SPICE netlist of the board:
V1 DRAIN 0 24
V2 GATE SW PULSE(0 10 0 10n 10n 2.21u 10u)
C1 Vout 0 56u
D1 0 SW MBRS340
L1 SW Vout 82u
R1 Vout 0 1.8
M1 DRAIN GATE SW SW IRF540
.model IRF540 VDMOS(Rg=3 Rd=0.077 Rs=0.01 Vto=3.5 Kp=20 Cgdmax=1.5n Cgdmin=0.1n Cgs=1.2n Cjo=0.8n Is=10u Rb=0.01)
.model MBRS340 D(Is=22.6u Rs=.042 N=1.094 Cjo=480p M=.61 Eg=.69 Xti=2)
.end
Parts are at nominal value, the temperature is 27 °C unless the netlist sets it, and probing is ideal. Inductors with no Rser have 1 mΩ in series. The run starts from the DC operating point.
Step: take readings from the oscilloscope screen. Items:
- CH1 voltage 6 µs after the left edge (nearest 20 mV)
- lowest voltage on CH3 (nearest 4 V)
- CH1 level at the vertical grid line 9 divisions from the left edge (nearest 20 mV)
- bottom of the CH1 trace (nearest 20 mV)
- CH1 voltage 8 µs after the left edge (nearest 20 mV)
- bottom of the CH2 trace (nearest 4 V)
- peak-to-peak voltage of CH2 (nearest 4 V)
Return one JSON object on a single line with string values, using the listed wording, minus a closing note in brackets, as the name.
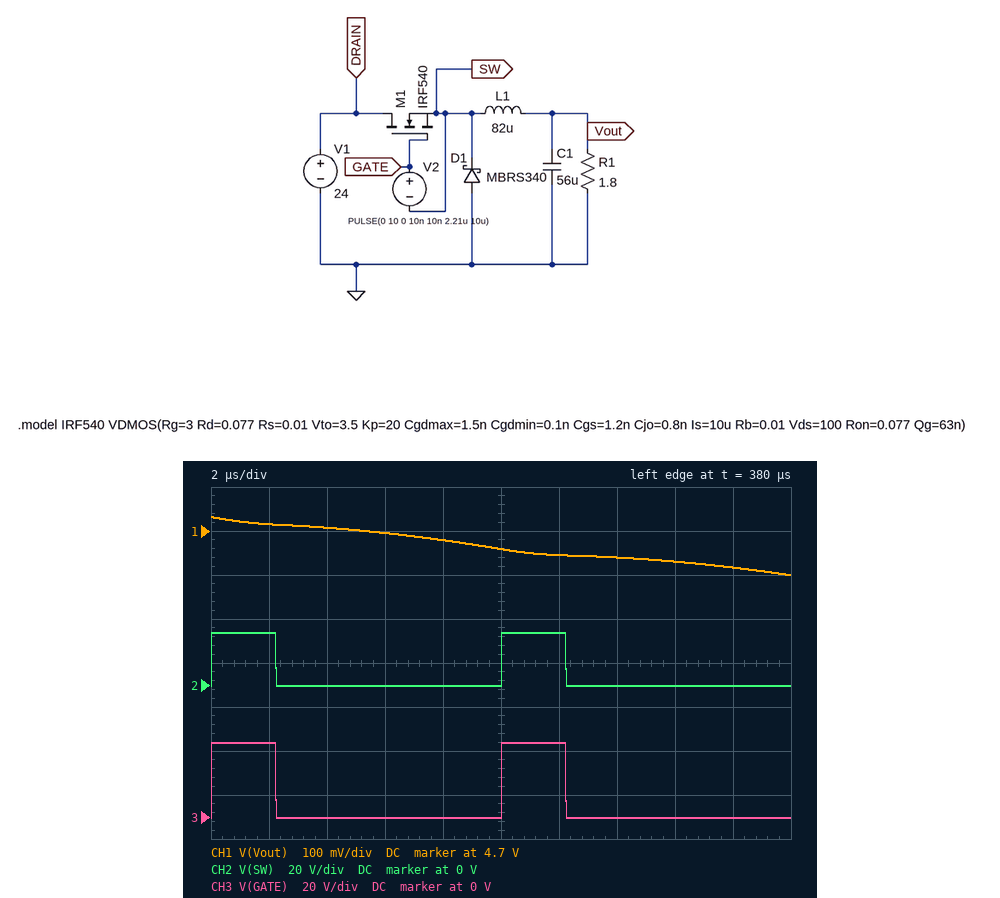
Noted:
{"CH1 voltage 6 µs after the left edge": "4.70 V", "lowest voltage on CH3": "0 V", "CH1 level at the vertical grid line 9 divisions from the left edge": "4.62 V", "bottom of the CH1 trace": "4.60 V", "CH1 voltage 8 µs after the left edge": "4.68 V", "bottom of the CH2 trace": "0 V", "peak-to-peak voltage of CH2": "24 V"}
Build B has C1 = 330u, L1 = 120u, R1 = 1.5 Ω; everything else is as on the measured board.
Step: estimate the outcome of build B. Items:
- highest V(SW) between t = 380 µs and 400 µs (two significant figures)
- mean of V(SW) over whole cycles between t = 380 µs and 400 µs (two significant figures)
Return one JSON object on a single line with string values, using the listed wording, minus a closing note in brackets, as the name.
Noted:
{"highest V(SW) between t = 380 µs and 400 µs": "23 V", "mean of V(SW) over whole cycles between t = 380 µs and 400 µs": "4.6 V"}
